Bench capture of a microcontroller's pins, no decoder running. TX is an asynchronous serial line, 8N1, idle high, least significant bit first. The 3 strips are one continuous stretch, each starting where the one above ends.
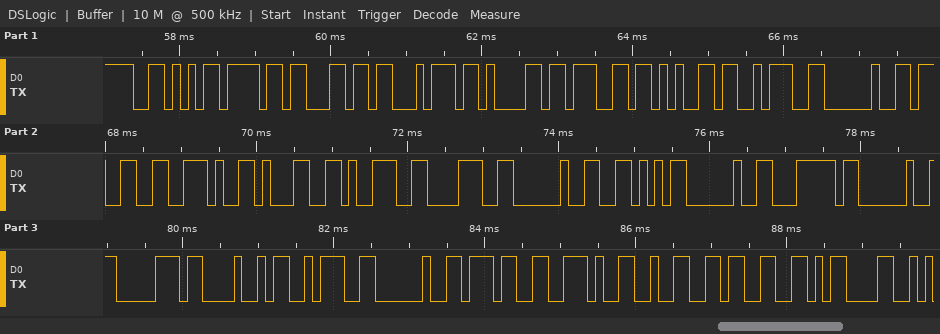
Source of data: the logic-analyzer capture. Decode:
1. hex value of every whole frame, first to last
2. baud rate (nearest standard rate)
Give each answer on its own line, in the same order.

56 6F 6C 74 61 67 65 3A 20 33 2E 31 39 38 20 56 20 7C 20 70 48 3A 20 37 2E 32 33 0D
9600 baud
